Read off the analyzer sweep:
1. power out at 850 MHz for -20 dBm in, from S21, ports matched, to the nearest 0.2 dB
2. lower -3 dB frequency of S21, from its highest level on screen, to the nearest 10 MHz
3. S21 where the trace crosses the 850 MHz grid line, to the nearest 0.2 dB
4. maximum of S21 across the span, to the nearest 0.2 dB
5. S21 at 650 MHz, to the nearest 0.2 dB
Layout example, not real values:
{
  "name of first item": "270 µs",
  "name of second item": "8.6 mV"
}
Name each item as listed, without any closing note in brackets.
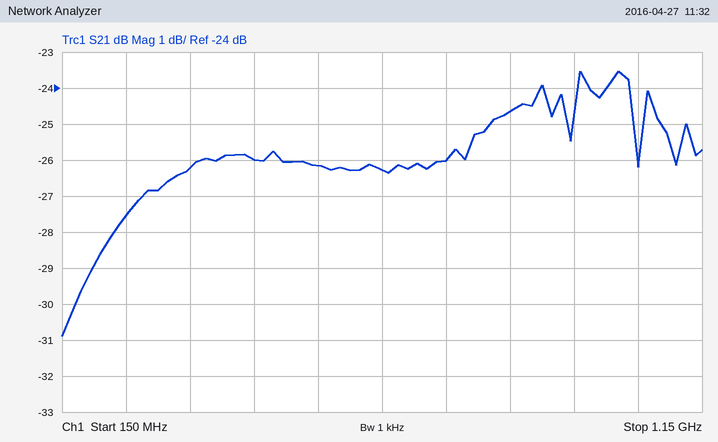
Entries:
{
  "power out at 850 MHz for -20 dBm in, from S21, ports matched, to the nearest 0.2 dB": "-44.6 dBm",
  "lower -3 dB frequency of S21, from its highest level on screen, to the nearest 10 MHz": "320 MHz",
  "S21 where the trace crosses the 850 MHz grid line, to the nearest 0.2 dB": "-24.6 dB",
  "maximum of S21 across the span, to the nearest 0.2 dB": "-23.6 dB",
  "S21 at 650 MHz, to the nearest 0.2 dB": "-26.2 dB"
}
